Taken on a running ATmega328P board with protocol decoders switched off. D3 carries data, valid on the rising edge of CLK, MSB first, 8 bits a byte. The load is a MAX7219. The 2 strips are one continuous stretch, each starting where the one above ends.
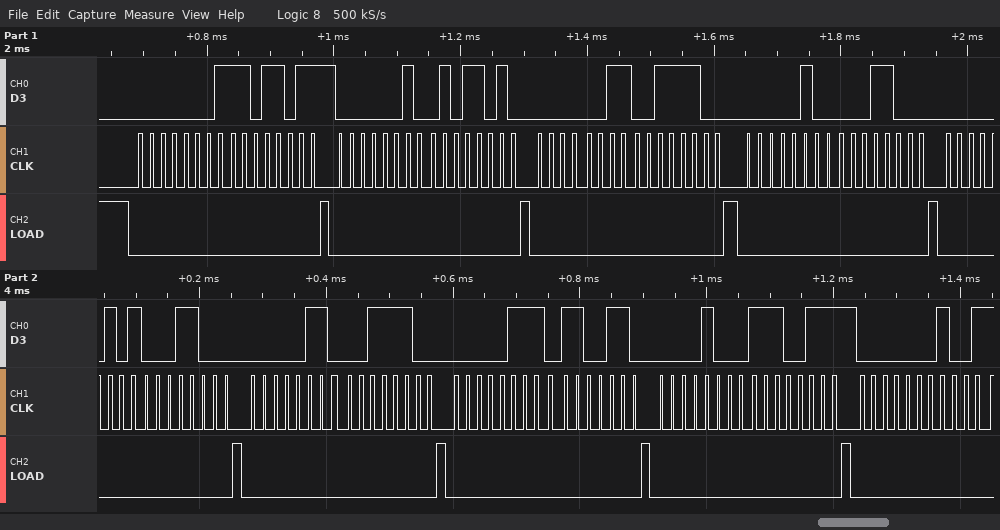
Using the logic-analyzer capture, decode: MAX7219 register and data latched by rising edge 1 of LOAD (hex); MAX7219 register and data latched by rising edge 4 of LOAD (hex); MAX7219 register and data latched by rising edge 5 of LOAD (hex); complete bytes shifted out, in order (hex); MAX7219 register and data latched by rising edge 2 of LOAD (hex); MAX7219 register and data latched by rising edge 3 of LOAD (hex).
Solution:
register 0x1, data 0xDB
register 0x4, data 0x18
register 0x5, data 0x18
01 DB 02 5A 03 3C 04 18 05 18 06 3C 07 66 08 E7 01
register 0x2, data 0x5A
register 0x3, data 0x3C
